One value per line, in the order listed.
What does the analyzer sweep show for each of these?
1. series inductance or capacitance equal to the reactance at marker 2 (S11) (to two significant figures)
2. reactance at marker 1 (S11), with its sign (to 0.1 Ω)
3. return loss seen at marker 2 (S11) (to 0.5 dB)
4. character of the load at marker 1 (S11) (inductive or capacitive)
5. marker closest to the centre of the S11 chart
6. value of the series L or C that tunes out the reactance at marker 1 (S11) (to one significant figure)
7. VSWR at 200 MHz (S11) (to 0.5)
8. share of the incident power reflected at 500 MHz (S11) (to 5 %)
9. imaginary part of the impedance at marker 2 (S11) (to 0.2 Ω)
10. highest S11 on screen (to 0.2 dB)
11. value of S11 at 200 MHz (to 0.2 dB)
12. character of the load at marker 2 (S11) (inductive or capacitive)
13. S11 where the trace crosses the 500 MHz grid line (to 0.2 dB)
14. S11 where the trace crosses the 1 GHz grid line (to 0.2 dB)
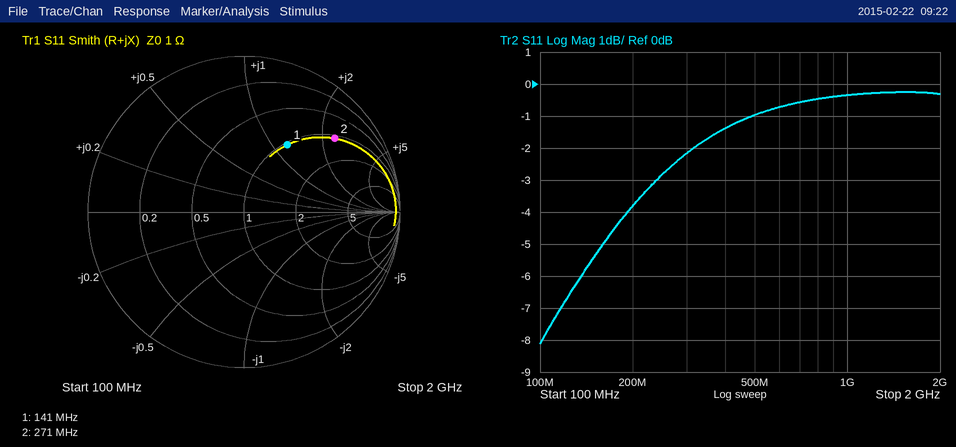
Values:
1.4 nH
+1.2 Ω
2.5 dB
inductive
marker 1
900 pF
4.5
80 %
+2.4 Ω
-0.2 dB
-3.8 dB
inductive
-1.0 dB
-0.4 dB
